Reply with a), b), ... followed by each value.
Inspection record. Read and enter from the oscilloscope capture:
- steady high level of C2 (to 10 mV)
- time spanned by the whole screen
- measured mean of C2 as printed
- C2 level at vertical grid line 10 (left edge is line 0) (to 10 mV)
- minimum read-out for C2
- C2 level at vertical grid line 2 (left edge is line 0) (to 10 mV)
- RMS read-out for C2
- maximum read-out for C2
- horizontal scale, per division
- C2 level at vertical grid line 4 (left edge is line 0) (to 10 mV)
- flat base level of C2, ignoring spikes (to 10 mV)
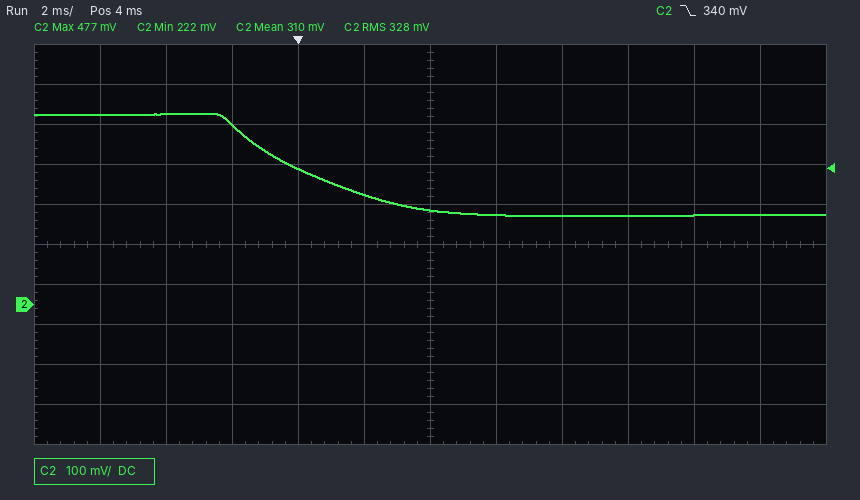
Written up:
a) 480 mV
b) 24 ms
c) 310 mV
d) 220 mV
e) 222 mV
f) 480 mV
g) 328 mV
h) 477 mV
i) 2 ms
j) 340 mV
k) 220 mV
